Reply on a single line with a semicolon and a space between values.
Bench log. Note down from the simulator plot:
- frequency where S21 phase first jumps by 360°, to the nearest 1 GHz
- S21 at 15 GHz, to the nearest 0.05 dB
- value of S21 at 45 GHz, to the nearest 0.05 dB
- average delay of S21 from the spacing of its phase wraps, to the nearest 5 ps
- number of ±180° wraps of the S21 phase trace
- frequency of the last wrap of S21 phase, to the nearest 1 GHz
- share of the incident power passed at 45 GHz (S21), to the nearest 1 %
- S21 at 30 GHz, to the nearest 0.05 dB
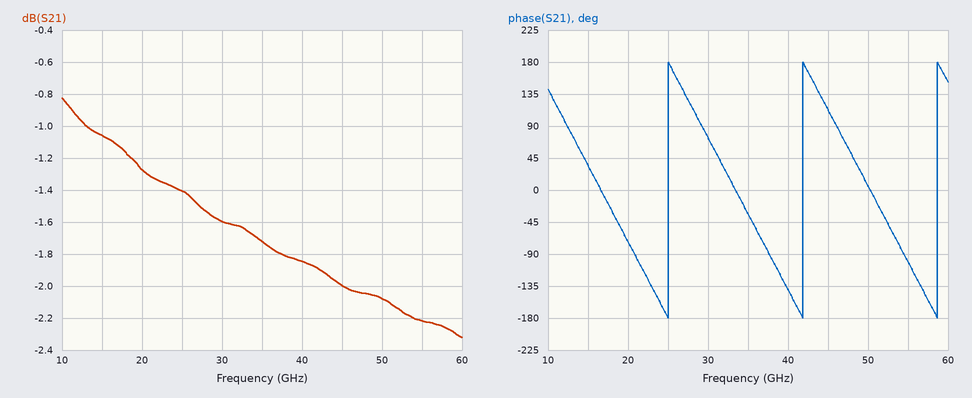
25 GHz; -1.05 dB; -2.00 dB; 60 ps; 3; 59 GHz; 63 %; -1.60 dB
